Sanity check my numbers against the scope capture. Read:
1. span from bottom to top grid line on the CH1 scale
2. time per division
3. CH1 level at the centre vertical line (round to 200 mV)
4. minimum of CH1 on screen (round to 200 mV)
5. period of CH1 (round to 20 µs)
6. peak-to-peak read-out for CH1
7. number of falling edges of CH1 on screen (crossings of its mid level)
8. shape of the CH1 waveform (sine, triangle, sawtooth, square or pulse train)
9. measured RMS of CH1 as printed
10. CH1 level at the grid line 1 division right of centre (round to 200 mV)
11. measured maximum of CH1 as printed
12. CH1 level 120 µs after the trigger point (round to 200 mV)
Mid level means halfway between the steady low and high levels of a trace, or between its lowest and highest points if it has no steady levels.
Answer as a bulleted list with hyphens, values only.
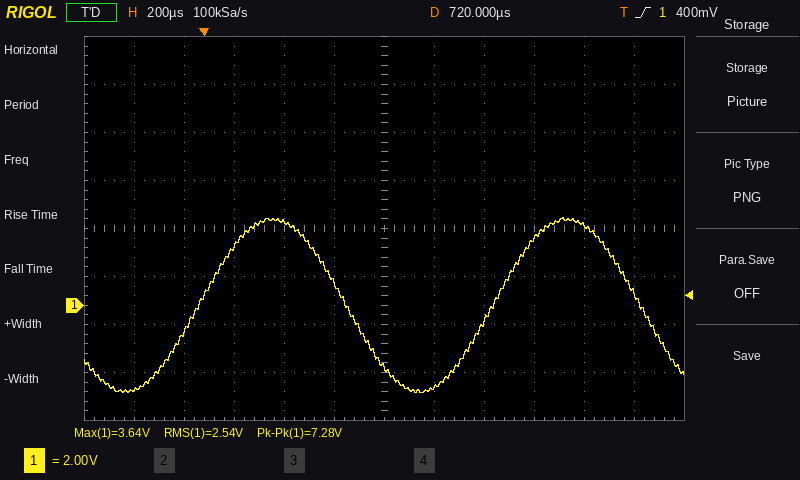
- 16 V
- 200 µs
- -2.6 V
- -3.6 V
- 1.18 ms
- 7.28 V
- 2
- sine
- 2.54 V
- -3.4 V
- 3.64 V
- 2.4 V
